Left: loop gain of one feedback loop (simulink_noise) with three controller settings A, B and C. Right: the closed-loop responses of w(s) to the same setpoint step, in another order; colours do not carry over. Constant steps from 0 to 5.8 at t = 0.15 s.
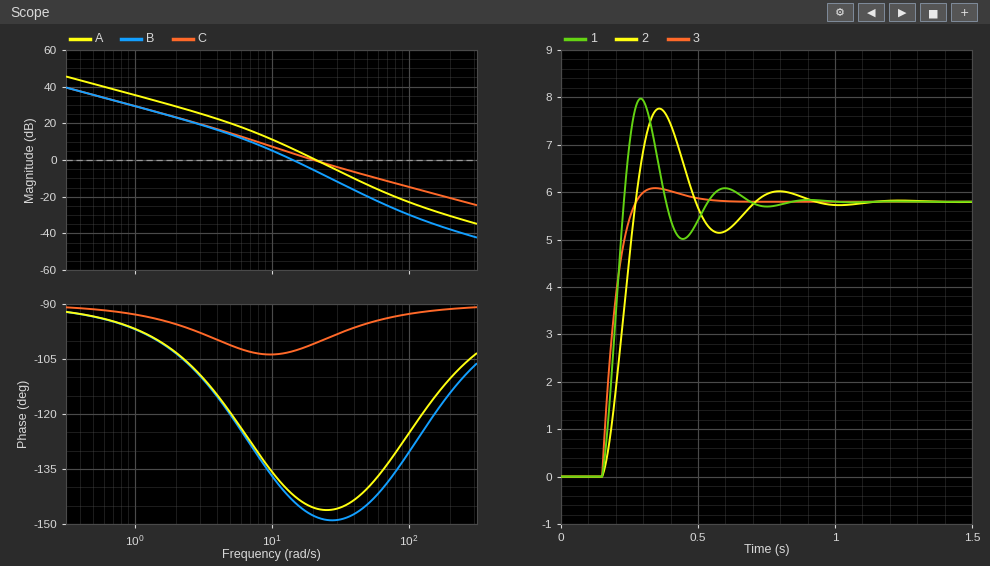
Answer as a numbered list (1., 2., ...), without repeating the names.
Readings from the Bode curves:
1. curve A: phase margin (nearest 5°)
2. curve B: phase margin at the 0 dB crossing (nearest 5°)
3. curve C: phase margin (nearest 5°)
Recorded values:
1. 35°
2. 35°
3. 80°
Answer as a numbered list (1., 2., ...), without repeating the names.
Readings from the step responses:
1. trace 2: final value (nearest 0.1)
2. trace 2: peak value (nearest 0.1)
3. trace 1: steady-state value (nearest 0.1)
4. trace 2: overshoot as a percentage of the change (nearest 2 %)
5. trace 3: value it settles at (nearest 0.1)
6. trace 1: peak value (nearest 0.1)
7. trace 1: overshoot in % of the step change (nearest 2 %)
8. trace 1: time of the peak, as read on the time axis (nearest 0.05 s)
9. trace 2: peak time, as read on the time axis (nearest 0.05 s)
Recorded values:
1. 5.8
2. 7.8
3. 5.8
4. 34 %
5. 5.8
6. 8.0
7. 38 %
8. 0.30 s
9. 0.35 s
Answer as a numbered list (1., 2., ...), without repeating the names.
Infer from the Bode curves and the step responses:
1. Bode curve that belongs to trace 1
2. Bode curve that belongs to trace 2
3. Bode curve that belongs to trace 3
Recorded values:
1. A
2. B
3. C
